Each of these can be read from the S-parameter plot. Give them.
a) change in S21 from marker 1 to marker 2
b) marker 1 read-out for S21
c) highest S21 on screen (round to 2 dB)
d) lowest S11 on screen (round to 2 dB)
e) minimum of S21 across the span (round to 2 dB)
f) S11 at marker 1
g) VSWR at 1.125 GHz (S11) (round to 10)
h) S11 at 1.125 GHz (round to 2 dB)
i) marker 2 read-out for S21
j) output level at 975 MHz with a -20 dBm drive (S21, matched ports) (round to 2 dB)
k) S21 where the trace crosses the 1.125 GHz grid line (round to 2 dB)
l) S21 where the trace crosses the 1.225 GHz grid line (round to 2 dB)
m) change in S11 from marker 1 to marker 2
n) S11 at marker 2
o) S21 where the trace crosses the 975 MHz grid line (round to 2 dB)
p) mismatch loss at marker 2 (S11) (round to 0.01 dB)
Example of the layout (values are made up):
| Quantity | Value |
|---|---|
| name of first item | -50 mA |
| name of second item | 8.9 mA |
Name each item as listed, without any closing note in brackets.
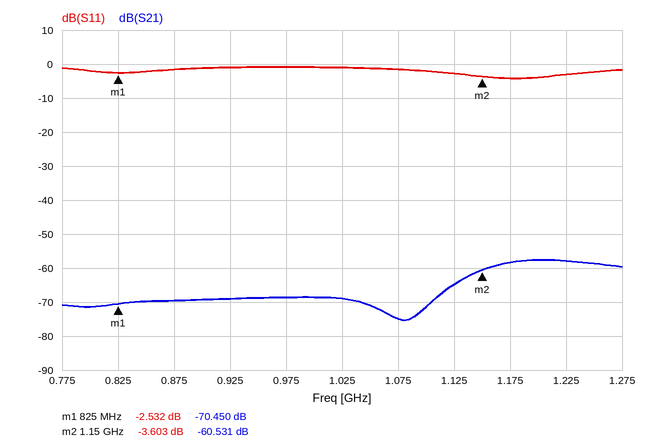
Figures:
| Quantity | Value |
|---|---|
| change in S21 from marker 1 to marker 2 | 9.919 dB |
| marker 1 read-out for S21 | -70.450 dB |
| highest S21 on screen | -58 dB |
| lowest S11 on screen | -4 dB |
| minimum of S21 across the span | -76 dB |
| S11 at marker 1 | -2.532 dB |
| VSWR at 1.125 GHz (S11) | 10 |
| S11 at 1.125 GHz | -2 dB |
| marker 2 read-out for S21 | -60.531 dB |
| output level at 975 MHz with a -20 dBm drive (S21, matched ports) | -88 dBm |
| S21 where the trace crosses the 1.125 GHz grid line | -64 dB |
| S21 where the trace crosses the 1.225 GHz grid line | -58 dB |
| change in S11 from marker 1 to marker 2 | -1.071 dB |
| S11 at marker 2 | -3.603 dB |
| S21 where the trace crosses the 975 MHz grid line | -68 dB |
| mismatch loss at marker 2 (S11) | 2.49 dB |
